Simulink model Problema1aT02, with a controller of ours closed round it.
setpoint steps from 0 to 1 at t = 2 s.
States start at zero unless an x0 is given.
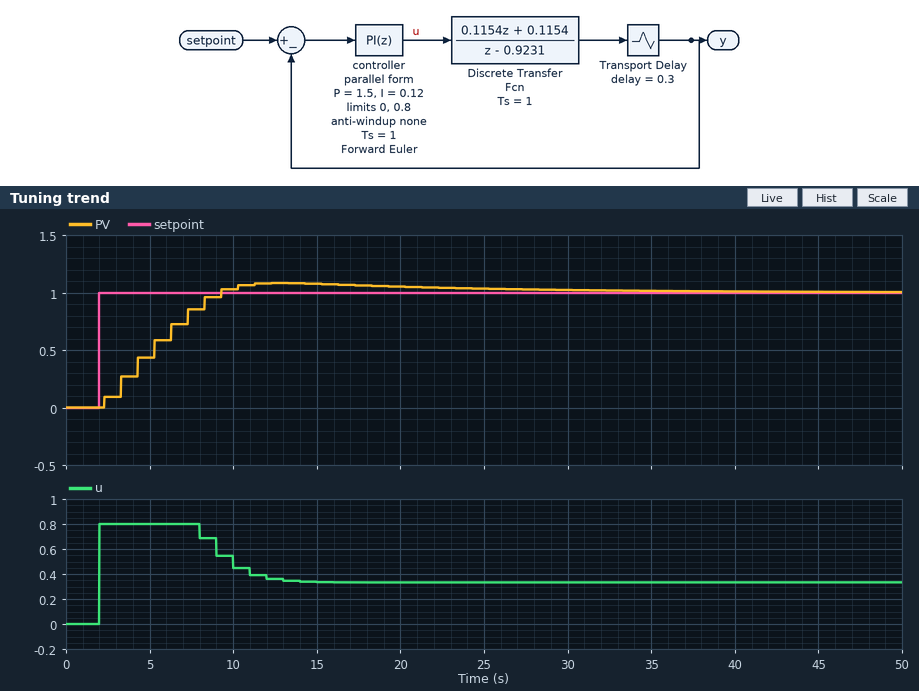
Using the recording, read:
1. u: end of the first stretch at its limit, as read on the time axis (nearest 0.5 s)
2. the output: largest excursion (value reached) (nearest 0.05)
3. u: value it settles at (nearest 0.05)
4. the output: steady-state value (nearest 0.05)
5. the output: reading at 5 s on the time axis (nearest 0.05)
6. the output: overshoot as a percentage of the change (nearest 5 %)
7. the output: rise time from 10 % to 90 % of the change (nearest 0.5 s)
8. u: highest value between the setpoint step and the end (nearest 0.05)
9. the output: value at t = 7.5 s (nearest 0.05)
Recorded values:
8.0 s
1.10
0.35
1.00
0.45
10 %
5.0 s
0.80
0.85
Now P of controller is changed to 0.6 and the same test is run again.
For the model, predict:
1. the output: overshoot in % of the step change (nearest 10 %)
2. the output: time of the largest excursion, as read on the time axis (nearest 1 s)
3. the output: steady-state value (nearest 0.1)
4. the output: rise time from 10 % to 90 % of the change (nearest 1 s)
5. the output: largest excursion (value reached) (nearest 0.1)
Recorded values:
20 %
17 s
1.0
6 s
1.2
